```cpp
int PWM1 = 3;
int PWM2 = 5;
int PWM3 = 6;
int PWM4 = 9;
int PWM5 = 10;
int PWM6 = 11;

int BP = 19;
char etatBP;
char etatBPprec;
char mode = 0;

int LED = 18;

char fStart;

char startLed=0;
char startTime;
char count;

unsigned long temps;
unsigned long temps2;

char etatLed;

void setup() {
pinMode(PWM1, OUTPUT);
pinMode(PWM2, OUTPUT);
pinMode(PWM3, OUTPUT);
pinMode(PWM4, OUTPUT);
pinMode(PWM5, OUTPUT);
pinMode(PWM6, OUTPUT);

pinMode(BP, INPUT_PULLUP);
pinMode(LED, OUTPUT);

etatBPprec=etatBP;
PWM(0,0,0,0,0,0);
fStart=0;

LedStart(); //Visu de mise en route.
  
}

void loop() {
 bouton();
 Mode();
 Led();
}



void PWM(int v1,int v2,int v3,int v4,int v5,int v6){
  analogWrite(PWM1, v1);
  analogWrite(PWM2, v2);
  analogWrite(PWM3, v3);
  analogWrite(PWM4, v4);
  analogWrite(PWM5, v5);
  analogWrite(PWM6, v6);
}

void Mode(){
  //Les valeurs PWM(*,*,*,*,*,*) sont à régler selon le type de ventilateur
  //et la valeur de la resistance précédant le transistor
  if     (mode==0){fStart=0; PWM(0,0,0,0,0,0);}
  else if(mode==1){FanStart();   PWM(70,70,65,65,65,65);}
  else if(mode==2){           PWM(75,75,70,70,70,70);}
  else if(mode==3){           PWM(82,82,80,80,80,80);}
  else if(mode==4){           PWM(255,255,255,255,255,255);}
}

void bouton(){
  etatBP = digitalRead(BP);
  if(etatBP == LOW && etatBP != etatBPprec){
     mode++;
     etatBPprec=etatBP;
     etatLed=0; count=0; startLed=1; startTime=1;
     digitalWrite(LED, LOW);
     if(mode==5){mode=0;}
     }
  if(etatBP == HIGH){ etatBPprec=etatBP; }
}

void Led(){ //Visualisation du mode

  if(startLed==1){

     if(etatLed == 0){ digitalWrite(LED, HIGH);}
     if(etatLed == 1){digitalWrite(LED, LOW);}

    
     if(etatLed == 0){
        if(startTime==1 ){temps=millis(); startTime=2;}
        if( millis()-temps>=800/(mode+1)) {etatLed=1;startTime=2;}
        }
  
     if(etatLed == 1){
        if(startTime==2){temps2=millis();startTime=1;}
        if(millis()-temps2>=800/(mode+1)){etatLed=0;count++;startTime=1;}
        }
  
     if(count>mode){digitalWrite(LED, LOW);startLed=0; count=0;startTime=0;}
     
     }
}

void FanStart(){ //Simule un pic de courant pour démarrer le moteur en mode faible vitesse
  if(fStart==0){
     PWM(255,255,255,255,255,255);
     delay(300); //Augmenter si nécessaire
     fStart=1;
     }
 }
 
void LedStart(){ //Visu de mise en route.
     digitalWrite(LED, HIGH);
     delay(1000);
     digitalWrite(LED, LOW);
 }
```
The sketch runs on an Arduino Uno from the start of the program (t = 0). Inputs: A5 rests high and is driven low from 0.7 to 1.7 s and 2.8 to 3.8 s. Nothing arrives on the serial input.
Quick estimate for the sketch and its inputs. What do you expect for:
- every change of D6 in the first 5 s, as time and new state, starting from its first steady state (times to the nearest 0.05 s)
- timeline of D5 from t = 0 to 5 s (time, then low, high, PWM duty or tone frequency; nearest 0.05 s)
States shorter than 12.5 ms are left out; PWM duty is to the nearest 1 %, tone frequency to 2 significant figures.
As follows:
0 s low; 2.8 s high; 3.1 s PWM 26 %
0 s low; 2.8 s high; 3.1 s PWM 28 %
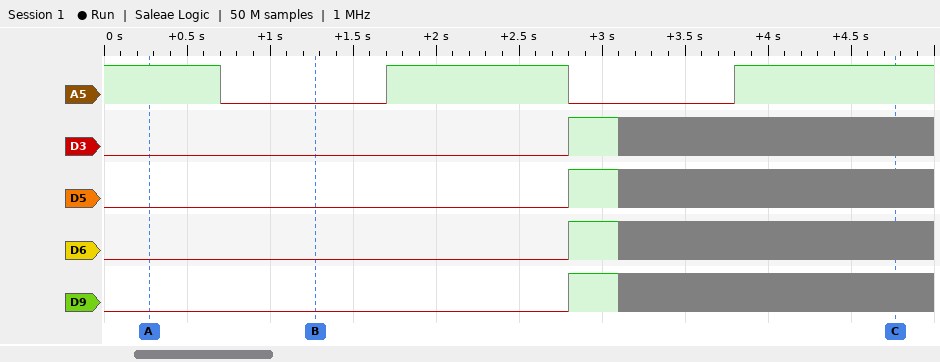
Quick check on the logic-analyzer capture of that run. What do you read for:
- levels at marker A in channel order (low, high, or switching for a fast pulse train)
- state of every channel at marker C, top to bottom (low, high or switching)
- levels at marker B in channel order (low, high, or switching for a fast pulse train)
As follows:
A5 high, D3 low, D5 low, D6 low, D9 low
A5 high, D3 switching, D5 switching, D6 switching, D9 switching
A5 low, D3 low, D5 low, D6 low, D9 low
